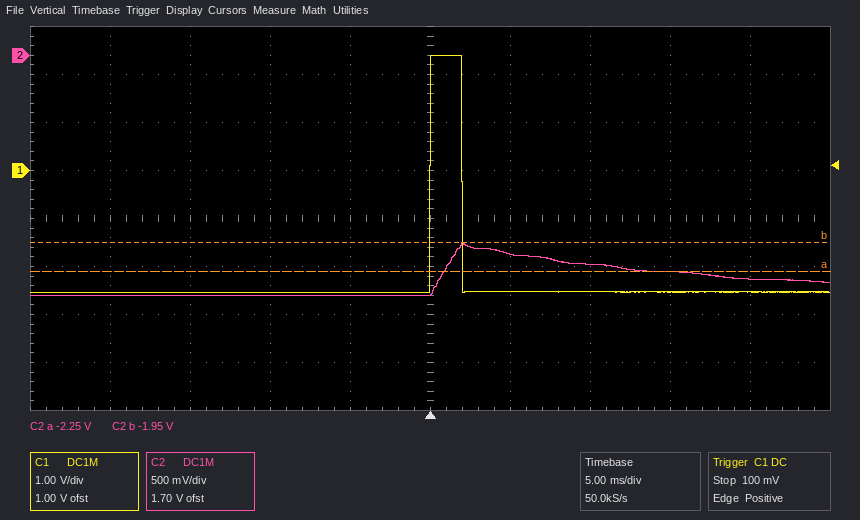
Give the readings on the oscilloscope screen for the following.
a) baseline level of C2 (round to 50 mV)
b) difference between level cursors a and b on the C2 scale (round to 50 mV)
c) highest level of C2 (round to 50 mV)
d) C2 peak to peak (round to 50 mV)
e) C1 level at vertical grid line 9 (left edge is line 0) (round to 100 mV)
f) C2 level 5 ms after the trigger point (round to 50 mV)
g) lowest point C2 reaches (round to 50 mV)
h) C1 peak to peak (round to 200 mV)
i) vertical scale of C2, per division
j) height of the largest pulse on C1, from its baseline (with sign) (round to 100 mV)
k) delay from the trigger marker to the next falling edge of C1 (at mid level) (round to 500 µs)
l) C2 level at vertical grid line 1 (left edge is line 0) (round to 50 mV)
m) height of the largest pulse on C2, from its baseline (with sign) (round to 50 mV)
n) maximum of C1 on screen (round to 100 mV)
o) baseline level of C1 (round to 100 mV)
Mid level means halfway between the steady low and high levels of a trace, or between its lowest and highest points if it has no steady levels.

-2.50 V
300 mV
-1.95 V
550 mV
-2.5 V
-2.05 V
-2.50 V
5.0 V
500 mV
+4.9 V
2.0 ms
-2.50 V
+550 mV
2.4 V
-2.5 V
